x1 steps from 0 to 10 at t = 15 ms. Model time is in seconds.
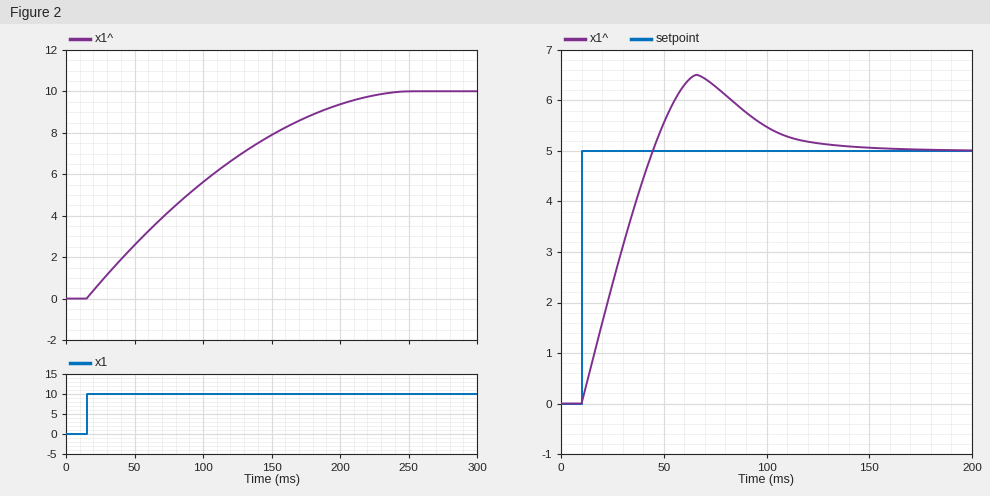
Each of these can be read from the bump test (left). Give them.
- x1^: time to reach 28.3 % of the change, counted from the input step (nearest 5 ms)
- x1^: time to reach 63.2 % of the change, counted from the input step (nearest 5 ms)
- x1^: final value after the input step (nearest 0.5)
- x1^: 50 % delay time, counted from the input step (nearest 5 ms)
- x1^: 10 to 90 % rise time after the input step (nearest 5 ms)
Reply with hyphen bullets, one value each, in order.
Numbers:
- 40 ms
- 100 ms
- 10.0
- 75 ms
- 155 ms
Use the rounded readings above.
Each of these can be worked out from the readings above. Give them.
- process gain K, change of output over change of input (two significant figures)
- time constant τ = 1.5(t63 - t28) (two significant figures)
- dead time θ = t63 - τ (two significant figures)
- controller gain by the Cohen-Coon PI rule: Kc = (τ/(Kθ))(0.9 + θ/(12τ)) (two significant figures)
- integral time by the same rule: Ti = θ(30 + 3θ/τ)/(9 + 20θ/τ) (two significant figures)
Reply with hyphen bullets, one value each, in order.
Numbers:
- 1.0
- 90 ms
- 10 ms
- 8.2
- 27 ms
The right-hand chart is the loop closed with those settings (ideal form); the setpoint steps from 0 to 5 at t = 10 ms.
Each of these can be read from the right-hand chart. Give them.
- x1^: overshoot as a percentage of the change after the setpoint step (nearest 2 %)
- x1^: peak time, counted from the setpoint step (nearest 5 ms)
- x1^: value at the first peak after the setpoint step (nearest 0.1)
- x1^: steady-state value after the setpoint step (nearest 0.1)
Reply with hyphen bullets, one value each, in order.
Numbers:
- 30 %
- 55 ms
- 6.5
- 5.0
